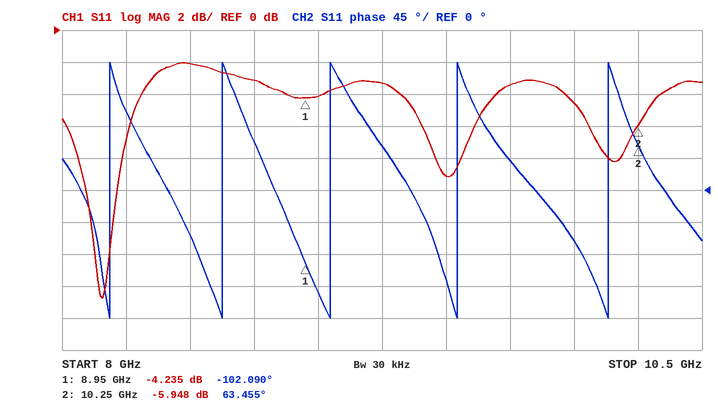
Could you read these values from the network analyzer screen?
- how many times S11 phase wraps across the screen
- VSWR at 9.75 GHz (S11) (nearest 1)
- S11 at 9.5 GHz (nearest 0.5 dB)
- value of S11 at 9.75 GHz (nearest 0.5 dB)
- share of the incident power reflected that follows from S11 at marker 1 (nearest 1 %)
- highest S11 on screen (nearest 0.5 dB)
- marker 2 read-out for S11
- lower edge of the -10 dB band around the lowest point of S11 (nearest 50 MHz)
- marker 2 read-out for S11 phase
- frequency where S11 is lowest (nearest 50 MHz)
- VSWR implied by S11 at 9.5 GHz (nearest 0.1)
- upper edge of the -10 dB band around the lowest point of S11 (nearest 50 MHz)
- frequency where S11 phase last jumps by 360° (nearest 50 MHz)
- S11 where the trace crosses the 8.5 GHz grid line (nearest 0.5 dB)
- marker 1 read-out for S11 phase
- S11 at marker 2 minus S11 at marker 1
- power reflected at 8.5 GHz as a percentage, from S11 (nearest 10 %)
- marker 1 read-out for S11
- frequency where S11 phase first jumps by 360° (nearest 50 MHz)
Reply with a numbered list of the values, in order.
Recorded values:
1. 5
2. 5
3. -9.0 dB
4. -3.5 dB
5. 38 %
6. -2.0 dB
7. -5.948 dB
8. 8.10 GHz
9. 63.455°
10. 8.15 GHz
11. 2.1
12. 8.20 GHz
13. 10.15 GHz
14. -2.0 dB
15. -102.090°
16. -1.713 dB
17. 60 %
18. -4.235 dB
19. 8.20 GHz
